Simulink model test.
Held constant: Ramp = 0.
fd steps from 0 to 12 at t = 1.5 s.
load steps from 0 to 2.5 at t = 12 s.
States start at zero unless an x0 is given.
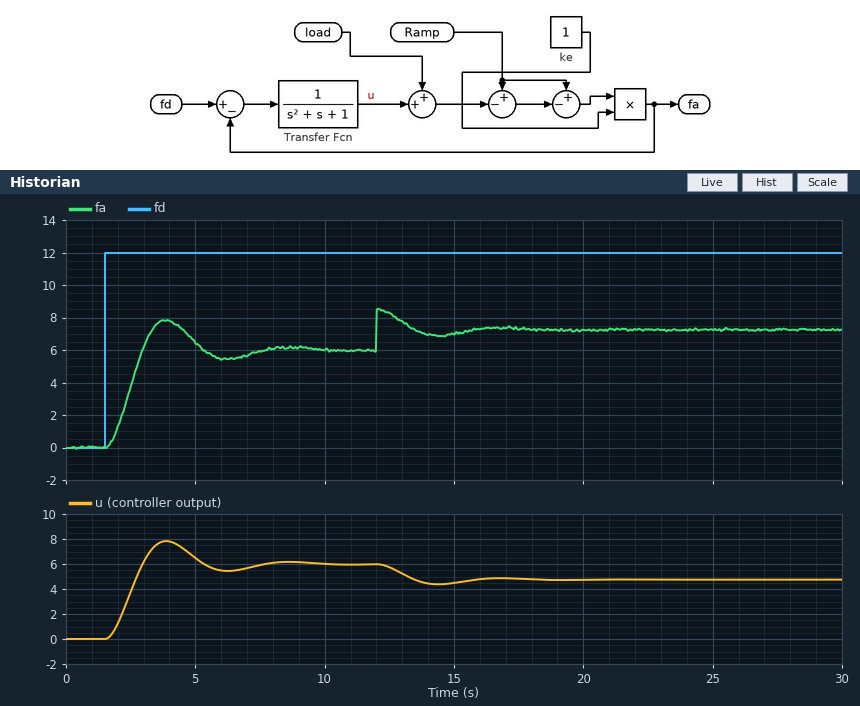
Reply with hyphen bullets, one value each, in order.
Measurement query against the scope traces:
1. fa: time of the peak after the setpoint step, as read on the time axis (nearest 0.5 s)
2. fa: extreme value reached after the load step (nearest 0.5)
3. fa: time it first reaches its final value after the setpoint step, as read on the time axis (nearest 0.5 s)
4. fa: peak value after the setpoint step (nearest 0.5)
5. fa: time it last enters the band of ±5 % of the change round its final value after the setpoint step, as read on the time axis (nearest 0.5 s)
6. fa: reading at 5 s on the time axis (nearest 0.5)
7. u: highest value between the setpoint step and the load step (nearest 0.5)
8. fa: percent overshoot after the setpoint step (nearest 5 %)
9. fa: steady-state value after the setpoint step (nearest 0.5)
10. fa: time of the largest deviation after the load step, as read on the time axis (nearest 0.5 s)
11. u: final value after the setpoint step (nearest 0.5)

- 4.0 s
- 8.5
- 3.0 s
- 8.0
- 7.0 s
- 6.5
- 8.0
- 30 %
- 6.0
- 12.0 s
- 6.0
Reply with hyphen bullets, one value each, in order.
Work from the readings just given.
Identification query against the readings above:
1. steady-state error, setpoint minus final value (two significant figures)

- 6.0
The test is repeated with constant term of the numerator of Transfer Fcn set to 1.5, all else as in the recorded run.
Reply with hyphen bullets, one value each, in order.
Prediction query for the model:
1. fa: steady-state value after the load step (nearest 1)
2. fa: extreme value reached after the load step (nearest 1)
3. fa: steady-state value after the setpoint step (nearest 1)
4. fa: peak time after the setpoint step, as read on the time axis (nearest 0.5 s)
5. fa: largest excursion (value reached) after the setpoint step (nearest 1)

- 8
- 10
- 7
- 3.5 s
- 10
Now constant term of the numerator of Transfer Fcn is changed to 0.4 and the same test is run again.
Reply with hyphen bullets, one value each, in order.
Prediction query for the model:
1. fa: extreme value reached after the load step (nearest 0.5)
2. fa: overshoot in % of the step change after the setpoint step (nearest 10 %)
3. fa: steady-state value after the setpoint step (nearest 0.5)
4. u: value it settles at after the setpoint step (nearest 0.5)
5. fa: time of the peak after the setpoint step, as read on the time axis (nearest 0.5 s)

- 6.0
- 20 %
- 3.5
- 3.5
- 4.5 s
